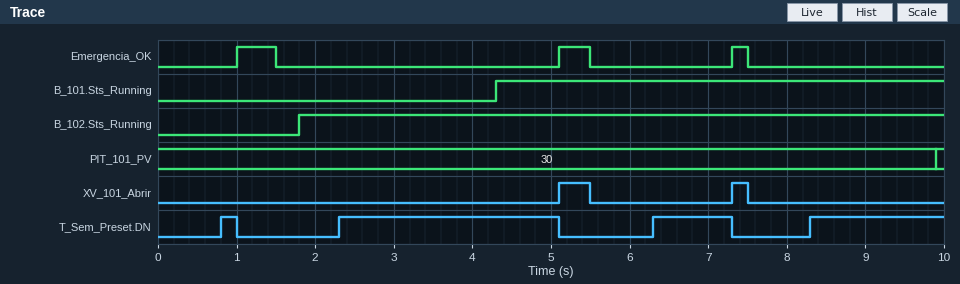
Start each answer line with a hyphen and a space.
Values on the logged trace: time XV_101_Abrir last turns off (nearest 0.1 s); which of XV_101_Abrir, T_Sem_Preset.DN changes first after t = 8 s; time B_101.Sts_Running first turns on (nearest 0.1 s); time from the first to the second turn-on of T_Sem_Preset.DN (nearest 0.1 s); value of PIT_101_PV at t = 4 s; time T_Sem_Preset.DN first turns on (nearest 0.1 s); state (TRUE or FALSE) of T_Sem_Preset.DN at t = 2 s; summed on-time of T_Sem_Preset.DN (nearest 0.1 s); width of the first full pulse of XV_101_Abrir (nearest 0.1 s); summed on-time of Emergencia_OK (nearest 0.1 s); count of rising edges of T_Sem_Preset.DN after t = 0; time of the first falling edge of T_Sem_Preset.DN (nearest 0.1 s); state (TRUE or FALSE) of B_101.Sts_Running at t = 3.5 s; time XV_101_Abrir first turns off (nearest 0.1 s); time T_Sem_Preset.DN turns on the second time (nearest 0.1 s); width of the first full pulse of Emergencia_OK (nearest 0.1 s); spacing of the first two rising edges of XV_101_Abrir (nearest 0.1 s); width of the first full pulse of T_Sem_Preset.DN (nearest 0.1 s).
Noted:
- 7.5 s
- T_Sem_Preset.DN
- 4.3 s
- 1.5 s
- 30
- 0.8 s
- FALSE
- 5.7 s
- 0.4 s
- 1.1 s
- 4
- 1.0 s
- FALSE
- 5.5 s
- 2.3 s
- 0.5 s
- 2.2 s
- 0.2 s
